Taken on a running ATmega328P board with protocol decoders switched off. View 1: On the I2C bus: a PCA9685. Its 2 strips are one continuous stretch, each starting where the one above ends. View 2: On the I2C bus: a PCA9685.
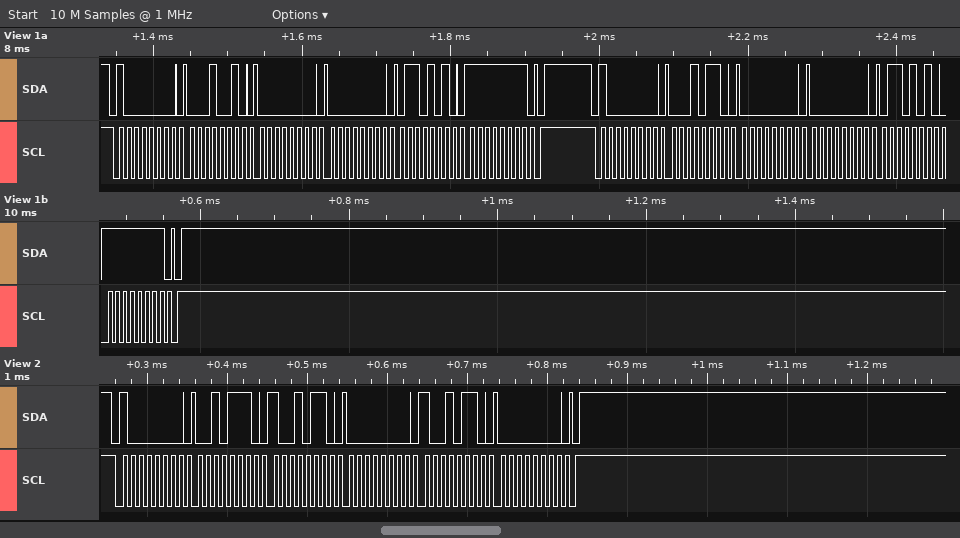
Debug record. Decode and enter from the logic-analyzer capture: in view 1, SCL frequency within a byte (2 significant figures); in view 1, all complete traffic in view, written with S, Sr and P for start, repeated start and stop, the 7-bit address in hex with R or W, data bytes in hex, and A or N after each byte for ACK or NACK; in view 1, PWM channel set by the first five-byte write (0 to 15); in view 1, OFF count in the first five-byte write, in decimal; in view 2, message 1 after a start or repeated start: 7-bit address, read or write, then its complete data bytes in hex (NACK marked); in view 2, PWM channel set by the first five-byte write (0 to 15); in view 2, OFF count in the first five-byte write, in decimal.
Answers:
100 kHz
S 40W A 12 A 00 A 00 A 6A A FF A P S 40W A 16 A 00 A 00 A 6A A FF A P
3
65386
0x40 write: 2E 96 00 96 00
10
150
